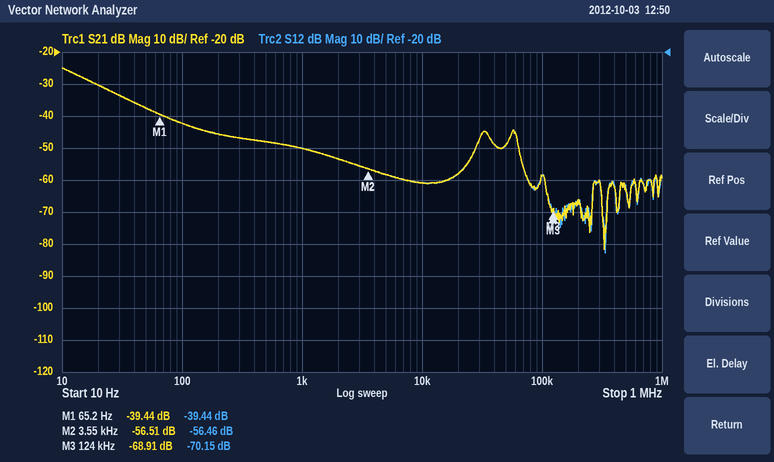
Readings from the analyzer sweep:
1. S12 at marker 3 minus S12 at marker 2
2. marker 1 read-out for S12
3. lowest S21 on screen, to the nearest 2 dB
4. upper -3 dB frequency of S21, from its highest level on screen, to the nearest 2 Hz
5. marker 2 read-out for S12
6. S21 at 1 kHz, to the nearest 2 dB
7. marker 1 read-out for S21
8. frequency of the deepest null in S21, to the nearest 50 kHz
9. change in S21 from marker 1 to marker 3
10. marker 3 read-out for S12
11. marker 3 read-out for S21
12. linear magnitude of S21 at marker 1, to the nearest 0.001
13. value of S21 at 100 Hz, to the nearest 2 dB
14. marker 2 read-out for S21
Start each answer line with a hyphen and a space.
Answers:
- -13.69 dB
- -39.44 dB
- -82 dB
- 14 Hz
- -56.46 dB
- -50 dB
- -39.44 dB
- 350 kHz
- -29.47 dB
- -70.15 dB
- -68.91 dB
- 0.011
- -42 dB
- -56.51 dB
